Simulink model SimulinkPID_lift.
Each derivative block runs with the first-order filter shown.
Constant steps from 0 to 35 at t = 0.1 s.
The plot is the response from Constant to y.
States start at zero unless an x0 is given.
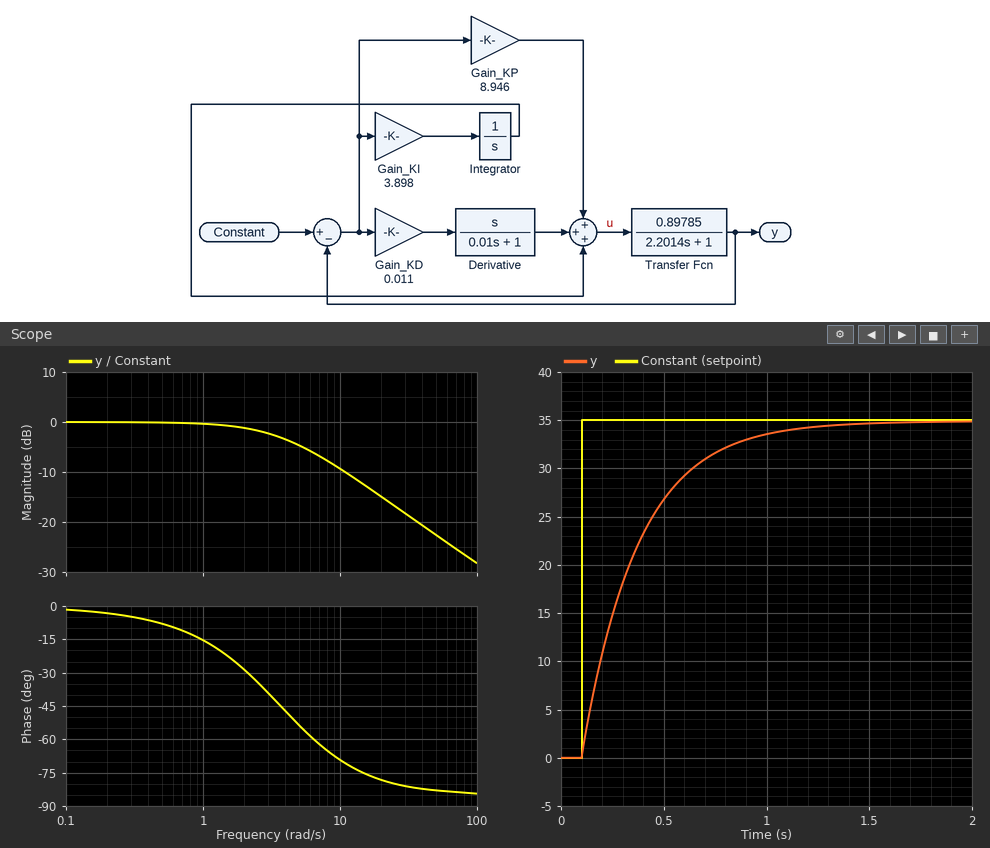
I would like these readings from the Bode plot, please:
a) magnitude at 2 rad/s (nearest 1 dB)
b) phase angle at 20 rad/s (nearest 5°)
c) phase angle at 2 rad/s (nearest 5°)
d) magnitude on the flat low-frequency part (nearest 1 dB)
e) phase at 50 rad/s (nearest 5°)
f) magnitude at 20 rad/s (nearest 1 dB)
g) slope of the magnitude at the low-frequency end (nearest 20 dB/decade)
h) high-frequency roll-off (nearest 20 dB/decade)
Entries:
-1 dB
-80°
-30°
0 dB
-85°
-15 dB
0 dB/decade
-20 dB/decade
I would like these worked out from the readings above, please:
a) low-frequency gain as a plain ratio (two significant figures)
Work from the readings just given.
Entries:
1.0
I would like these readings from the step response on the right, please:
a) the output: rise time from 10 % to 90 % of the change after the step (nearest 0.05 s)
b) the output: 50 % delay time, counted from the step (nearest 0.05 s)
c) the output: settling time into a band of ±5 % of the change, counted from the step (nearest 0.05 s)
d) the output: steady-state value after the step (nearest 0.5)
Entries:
0.60 s
0.20 s
0.85 s
35.0
